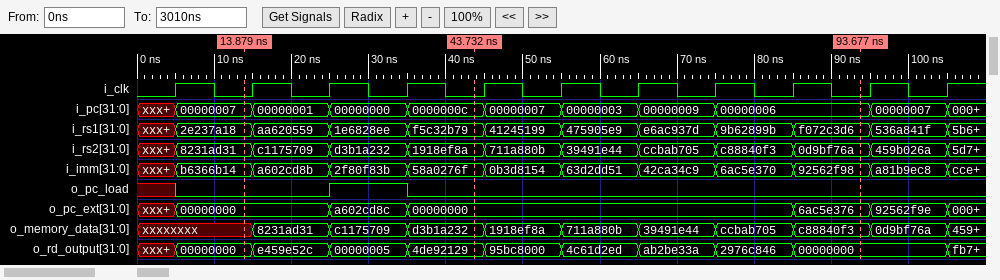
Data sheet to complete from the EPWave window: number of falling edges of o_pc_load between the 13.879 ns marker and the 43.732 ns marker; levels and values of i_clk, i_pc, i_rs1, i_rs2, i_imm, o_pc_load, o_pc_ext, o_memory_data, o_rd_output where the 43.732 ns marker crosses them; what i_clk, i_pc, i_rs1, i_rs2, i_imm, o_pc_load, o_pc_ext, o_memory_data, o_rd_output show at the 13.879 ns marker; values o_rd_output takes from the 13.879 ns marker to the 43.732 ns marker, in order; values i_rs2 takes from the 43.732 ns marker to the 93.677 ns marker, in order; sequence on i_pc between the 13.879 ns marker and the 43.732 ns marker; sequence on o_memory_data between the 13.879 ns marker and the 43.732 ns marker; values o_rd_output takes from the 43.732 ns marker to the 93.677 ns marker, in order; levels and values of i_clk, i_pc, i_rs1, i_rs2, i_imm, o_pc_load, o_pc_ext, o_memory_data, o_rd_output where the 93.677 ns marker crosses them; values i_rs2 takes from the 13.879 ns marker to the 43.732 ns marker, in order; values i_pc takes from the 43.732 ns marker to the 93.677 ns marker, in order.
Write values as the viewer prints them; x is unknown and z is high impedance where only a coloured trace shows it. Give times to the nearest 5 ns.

1
i_clk=0, i_pc=0000000c, i_rs1=f5c32b79, i_rs2=1918ef8a, i_imm=58a0276f, o_pc_load=0, o_pc_ext=00000000, o_memory_data=d3b1a232, o_rd_output=4de92129
i_clk=0, i_pc=00000007, i_rs1=2e237a18, i_rs2=8231ad31, i_imm=b6366b14, o_pc_load=0, o_pc_ext=00000000, o_memory_data=xxxxxxxx, o_rd_output=00000000
00000000, e459e52c, 00000005, 4de92129
1918ef8a, 711a880b, 39491e44, ccbab705, c88840f3, 0d9bf76a
00000007, 00000001, 00000000, 0000000c
xxxxxxxx, 8231ad31, c1175709, d3b1a232
4de92129, 95bc8000, 4c61d2ed, ab2be33a, 2976c846, 00000000
i_clk=0, i_pc=00000006, i_rs1=f072c3d6, i_rs2=0d9bf76a, i_imm=92562f98, o_pc_load=0, o_pc_ext=6ac5e376, o_memory_data=c88840f3, o_rd_output=00000000
8231ad31, c1175709, d3b1a232, 1918ef8a
0000000c, 00000007, 00000003, 00000009, 00000006
